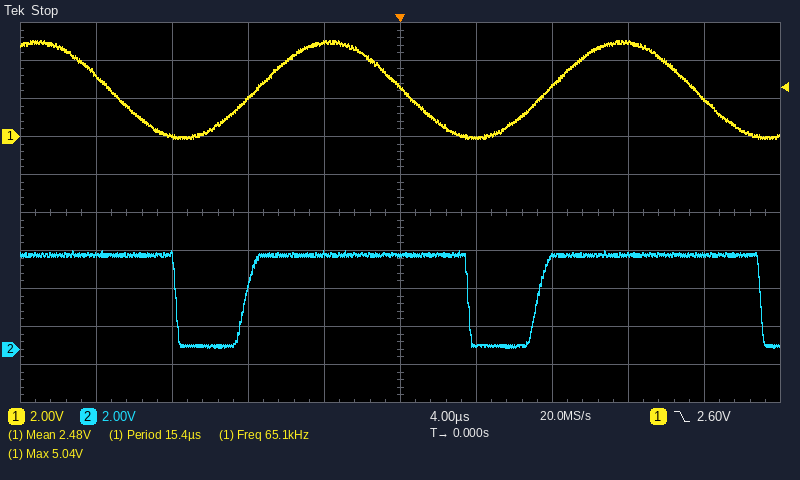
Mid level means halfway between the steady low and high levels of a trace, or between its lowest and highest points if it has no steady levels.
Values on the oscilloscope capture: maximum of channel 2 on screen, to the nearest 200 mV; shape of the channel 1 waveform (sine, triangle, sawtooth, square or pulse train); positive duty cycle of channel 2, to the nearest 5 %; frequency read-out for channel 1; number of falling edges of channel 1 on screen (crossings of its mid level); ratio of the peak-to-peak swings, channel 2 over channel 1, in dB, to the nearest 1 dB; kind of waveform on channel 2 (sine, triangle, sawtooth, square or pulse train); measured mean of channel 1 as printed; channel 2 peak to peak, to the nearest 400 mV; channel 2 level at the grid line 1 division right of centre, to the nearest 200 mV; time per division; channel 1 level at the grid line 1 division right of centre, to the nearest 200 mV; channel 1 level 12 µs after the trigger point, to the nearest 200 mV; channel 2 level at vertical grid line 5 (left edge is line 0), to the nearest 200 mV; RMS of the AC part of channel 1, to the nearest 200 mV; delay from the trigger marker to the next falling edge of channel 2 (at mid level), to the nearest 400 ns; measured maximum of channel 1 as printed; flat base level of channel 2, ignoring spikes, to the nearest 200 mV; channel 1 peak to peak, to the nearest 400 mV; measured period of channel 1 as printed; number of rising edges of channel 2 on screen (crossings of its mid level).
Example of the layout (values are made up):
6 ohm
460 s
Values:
5.2 V
sine
75 %
65.1 kHz
3
0 dB
pulse train
2.48 V
5.2 V
200 mV
4 µs
0.0 V
5.0 V
5.0 V
1.8 V
3.6 µs
5.04 V
200 mV
5.2 V
15.4 µs
2
